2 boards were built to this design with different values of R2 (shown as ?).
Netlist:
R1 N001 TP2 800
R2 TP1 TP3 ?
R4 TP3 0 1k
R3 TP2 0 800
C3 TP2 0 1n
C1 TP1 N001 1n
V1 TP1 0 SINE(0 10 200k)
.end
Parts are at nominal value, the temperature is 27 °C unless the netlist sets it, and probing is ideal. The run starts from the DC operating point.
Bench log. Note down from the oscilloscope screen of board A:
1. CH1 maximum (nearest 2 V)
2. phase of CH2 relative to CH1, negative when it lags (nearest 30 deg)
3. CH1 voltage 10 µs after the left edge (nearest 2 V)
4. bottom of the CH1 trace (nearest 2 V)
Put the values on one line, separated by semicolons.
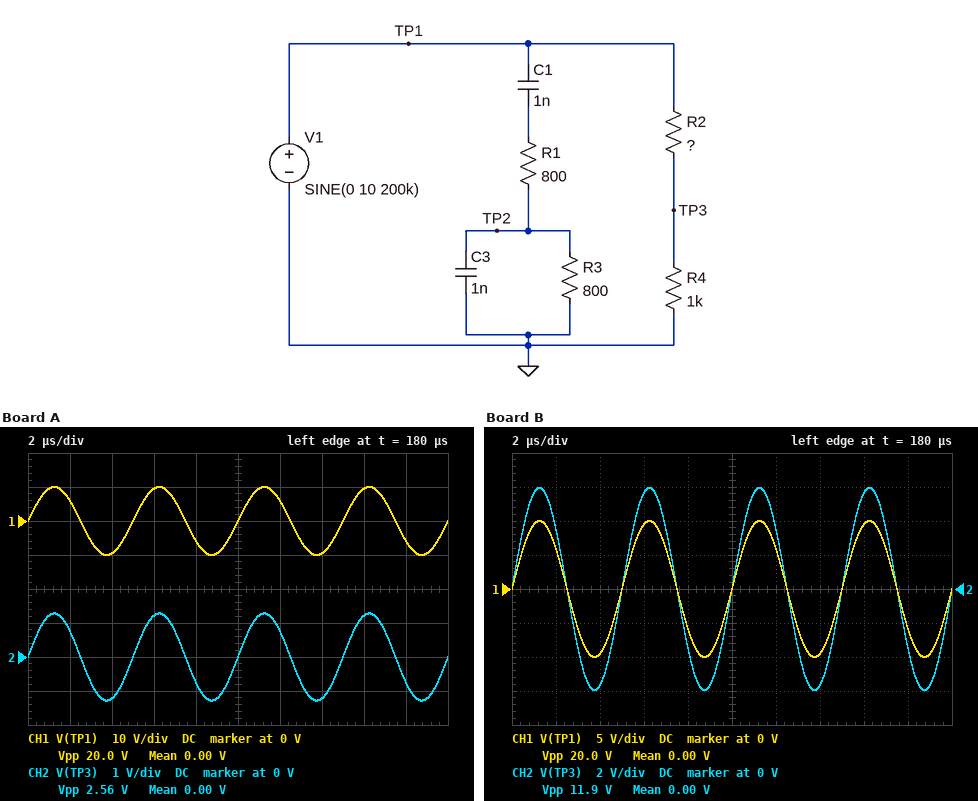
10 V; 0 deg; 0 V; -10 V
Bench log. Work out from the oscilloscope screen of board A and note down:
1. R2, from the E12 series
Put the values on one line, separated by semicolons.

6.8 kΩ
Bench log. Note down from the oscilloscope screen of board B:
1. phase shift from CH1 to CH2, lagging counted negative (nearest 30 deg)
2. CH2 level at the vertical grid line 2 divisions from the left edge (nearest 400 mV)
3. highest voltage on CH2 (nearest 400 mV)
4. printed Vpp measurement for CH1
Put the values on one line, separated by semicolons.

0 deg; -5.6 V; 6.0 V; 20.0 V
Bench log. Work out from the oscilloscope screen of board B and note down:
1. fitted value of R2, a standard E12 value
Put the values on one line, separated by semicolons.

680 Ω
